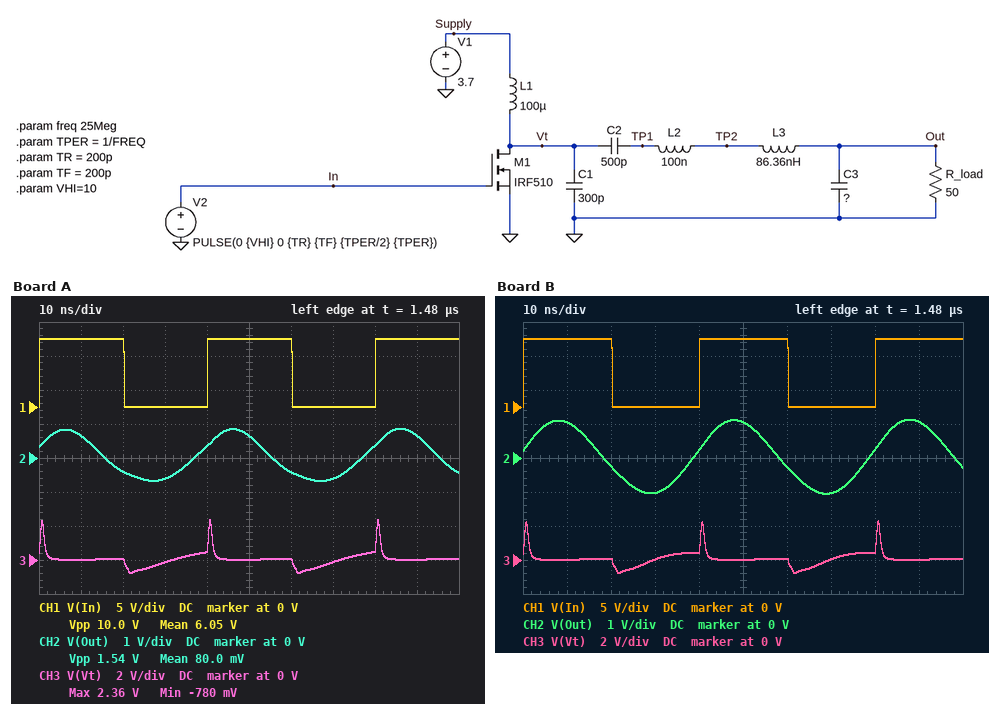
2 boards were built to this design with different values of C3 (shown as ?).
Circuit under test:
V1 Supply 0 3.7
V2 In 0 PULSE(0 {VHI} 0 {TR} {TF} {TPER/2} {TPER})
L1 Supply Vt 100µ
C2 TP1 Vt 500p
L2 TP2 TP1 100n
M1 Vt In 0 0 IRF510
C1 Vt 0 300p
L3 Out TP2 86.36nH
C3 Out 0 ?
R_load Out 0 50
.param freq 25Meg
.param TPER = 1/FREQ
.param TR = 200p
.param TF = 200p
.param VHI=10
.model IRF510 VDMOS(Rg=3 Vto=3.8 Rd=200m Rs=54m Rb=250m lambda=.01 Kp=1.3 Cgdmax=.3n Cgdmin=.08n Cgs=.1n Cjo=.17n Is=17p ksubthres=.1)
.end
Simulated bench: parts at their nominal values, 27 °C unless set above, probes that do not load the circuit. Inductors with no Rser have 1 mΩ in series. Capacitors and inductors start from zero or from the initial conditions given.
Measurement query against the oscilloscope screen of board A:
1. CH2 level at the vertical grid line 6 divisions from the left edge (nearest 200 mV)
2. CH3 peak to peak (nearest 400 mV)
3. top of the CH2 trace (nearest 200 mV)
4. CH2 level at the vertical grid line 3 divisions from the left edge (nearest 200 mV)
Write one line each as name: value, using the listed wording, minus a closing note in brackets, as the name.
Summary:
CH2 level at the vertical grid line 6 divisions from the left edge: -400 mV
CH3 peak to peak: 3.2 V
top of the CH2 trace: 800 mV
CH2 level at the vertical grid line 3 divisions from the left edge: -600 mV
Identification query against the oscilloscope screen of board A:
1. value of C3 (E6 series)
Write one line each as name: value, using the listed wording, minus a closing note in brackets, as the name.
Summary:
value of C3: 220 pF
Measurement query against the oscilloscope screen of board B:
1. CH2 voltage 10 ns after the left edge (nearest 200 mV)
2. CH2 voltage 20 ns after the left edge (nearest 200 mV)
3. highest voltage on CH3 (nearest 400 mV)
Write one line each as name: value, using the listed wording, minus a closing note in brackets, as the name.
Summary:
CH2 voltage 10 ns after the left edge: 1.0 V
CH2 voltage 20 ns after the left edge: -200 mV
highest voltage on CH3: 2.4 V
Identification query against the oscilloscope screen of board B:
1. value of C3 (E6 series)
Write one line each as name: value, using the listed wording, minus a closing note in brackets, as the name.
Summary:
value of C3: 330 pF
